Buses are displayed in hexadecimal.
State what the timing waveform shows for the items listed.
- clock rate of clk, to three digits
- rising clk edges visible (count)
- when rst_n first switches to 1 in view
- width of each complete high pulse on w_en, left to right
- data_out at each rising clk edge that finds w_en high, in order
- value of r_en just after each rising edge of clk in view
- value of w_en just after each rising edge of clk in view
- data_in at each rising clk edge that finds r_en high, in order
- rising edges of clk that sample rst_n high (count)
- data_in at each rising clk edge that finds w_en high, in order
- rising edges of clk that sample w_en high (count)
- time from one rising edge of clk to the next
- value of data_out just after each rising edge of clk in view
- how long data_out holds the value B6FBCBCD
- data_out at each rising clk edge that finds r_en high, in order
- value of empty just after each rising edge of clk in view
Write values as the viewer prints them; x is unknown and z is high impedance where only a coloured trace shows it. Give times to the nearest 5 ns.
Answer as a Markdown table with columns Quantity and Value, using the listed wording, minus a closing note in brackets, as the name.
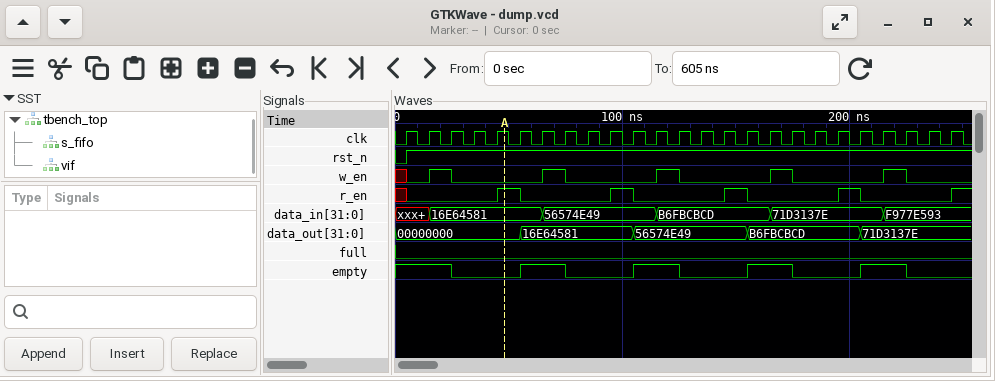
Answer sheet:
| Quantity | Value |
|---|---|
| clock rate of clk, to three digits | 100 MHz |
| rising clk edges visible | 25 |
| when rst_n first switches to 1 in view | 5 ns |
| width of each complete high pulse on w_en, left to right | 10 ns, 10 ns, 10 ns, 10 ns, 10 ns |
| data_out at each rising clk edge that finds w_en high, in order | 00000000, 16E64581, 56574E49, B6FBCBCD, 71D3137E |
| value of r_en just after each rising edge of clk in view | 0 0 0 0 1 0 0 0 0 1 0 0 0 0 1 0 0 0 0 1 0 0 0 0 1 |
| value of w_en just after each rising edge of clk in view | 0 1 0 0 0 0 1 0 0 0 0 1 0 0 0 0 1 0 0 0 0 1 0 0 0 |
| data_in at each rising clk edge that finds r_en high, in order | 16E64581, 56574E49, B6FBCBCD, 71D3137E |
| rising edges of clk that sample rst_n high | 24 |
| data_in at each rising clk edge that finds w_en high, in order | 16E64581, 56574E49, B6FBCBCD, 71D3137E, F977E593 |
| rising edges of clk that sample w_en high | 5 |
| time from one rising edge of clk to the next | 10 ns |
| value of data_out just after each rising edge of clk in view | 00000000, 00000000, 00000000, 00000000, 00000000, 16E64581, 16E64581, 16E64581, 16E64581, 16E64581, 56574E49, 56574E49, 56574E49, 56574E49, 56574E49, B6FBCBCD, B6FBCBCD, B6FBCBCD, B6FBCBCD, B6FBCBCD, 71D3137E, 71D3137E, 71D3137E, 71D3137E, 71D3137E |
| how long data_out holds the value B6FBCBCD | 50 ns |
| data_out at each rising clk edge that finds r_en high, in order | 00000000, 16E64581, 56574E49, B6FBCBCD |
| value of empty just after each rising edge of clk in view | 1 1 0 0 0 1 1 0 0 0 1 1 0 0 0 1 1 0 0 0 1 1 0 0 0 |
